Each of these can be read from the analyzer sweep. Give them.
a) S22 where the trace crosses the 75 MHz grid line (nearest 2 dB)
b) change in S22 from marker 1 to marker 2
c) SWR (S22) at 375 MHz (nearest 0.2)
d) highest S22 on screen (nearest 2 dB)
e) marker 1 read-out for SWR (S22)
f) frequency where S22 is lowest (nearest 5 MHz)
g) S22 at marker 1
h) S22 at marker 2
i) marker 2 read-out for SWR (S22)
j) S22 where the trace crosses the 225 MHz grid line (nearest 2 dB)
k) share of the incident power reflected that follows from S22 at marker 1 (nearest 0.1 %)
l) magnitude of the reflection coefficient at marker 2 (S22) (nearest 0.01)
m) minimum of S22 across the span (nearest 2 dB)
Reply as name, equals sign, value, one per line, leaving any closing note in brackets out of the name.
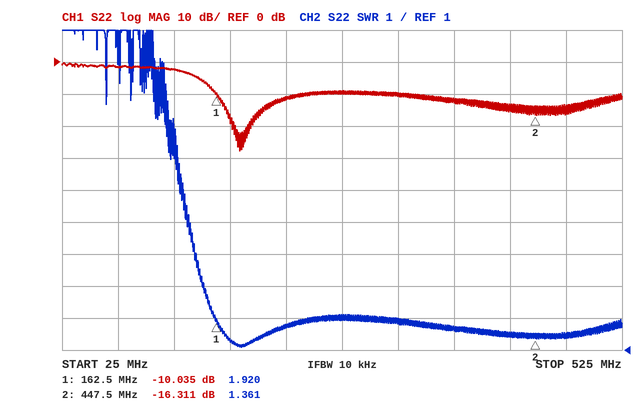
S22 where the trace crosses the 75 MHz grid line = -2 dB
change in S22 from marker 1 to marker 2 = -6.276 dB
SWR (S22) at 375 MHz = 1.6
highest S22 on screen = 0 dB
marker 1 read-out for SWR = 1.920
frequency where S22 is lowest = 185 MHz
S22 at marker 1 = -10.035 dB
S22 at marker 2 = -16.311 dB
marker 2 read-out for SWR = 1.361
S22 where the trace crosses the 225 MHz grid line = -12 dB
share of the incident power reflected that follows from S22 at marker 1 = 9.9 %
magnitude of the reflection coefficient at marker 2 (S22) = 0.15
minimum of S22 across the span = -28 dB
